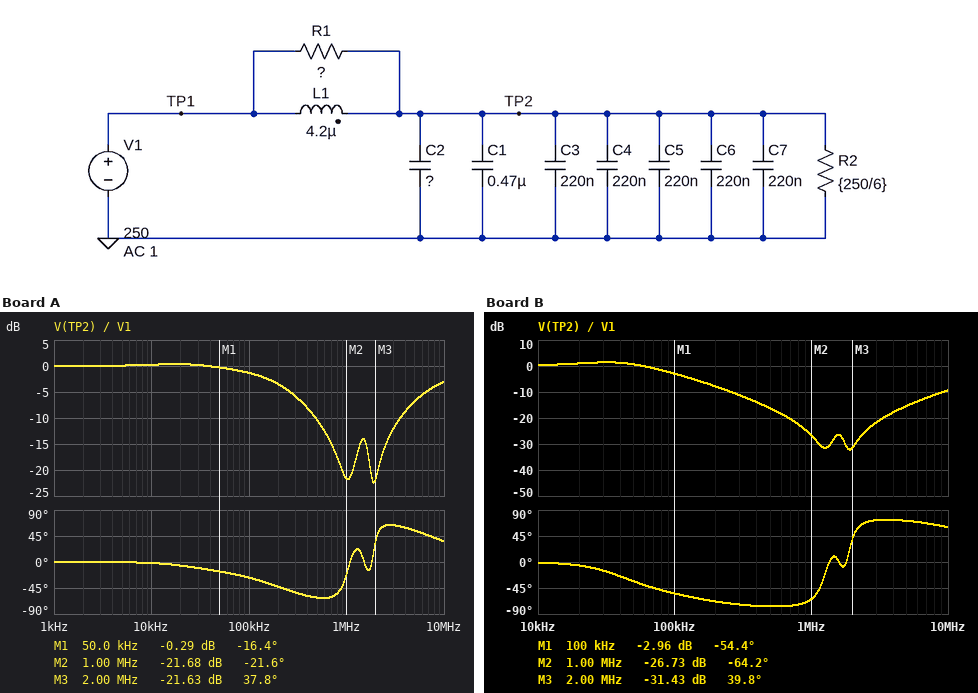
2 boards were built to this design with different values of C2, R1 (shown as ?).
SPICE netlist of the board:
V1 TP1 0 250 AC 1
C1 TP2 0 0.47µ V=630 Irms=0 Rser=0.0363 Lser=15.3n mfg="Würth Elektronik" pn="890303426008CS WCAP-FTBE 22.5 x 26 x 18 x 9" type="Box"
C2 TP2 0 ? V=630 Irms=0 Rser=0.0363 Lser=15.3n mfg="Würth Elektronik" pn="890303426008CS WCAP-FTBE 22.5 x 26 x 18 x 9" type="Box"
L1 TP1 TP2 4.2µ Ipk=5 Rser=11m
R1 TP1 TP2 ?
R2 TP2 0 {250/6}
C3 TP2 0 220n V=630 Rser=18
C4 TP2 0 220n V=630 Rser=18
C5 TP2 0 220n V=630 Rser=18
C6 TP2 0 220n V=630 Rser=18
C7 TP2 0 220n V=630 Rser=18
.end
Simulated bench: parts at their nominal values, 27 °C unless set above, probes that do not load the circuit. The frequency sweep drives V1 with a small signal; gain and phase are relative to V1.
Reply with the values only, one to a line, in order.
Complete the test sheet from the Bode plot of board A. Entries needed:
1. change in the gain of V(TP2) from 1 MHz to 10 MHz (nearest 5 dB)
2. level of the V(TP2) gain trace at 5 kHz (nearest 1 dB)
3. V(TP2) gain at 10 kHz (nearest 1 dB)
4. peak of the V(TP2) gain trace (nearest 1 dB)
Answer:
20 dB
0 dB
0 dB
0 dB
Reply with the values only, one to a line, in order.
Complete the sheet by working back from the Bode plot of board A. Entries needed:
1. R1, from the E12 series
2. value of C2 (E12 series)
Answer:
0.39 Ω
1.5 µF
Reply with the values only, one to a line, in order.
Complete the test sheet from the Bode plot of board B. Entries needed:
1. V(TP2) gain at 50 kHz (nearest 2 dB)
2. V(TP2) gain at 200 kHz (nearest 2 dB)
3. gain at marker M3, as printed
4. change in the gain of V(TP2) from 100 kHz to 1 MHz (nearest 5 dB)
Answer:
0 dB
-8 dB
-31.43 dB
-25 dB
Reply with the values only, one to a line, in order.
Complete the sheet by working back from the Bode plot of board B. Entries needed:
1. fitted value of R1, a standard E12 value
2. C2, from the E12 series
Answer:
1.2 Ω
1 µF
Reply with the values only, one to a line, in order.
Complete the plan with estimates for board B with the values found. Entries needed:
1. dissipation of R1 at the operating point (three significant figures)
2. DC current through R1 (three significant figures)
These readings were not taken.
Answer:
3.56 mW
54.5 mA
